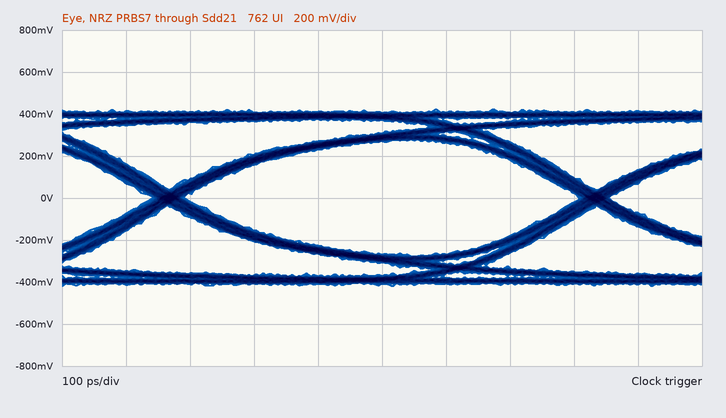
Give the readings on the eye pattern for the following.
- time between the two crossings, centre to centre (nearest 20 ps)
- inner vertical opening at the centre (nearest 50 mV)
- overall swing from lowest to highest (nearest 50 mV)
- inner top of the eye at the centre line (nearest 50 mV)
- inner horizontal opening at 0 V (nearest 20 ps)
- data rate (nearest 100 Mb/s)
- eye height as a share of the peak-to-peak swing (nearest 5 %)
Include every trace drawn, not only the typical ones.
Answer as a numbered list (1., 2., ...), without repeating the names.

1. 660 ps
2. 550 mV
3. 850 mV
4. 250 mV
5. 620 ps
6. 1.5 Gb/s
7. 65 %
